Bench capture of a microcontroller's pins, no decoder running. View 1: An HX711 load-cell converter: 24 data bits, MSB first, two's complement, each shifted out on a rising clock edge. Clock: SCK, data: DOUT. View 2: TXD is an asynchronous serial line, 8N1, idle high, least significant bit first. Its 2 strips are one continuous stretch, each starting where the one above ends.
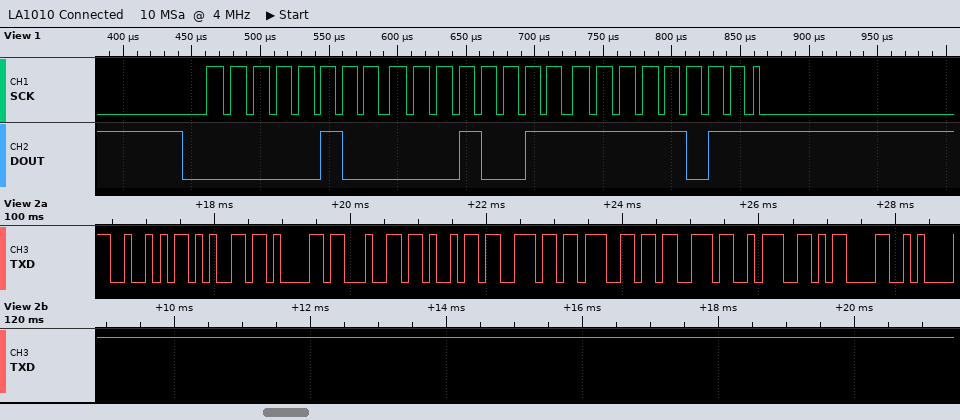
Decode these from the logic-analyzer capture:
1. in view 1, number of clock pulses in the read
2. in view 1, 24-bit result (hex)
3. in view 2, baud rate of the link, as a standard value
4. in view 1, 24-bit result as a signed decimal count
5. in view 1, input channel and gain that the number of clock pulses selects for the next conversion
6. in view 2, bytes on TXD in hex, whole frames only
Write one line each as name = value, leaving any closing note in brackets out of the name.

in view 1, number of clock pulses in the read = 25
in view 1, 24-bit result = 0x0413FB
in view 2, baud rate of the link, as a standard value = 9600 baud
in view 1, 24-bit result as a signed decimal count = 267259
in view 1, input channel and gain that the number of clock pulses selects for the next conversion = channel A, gain 128
in view 2, bytes on TXD in hex, whole frames only = 52 65 61 64 69 6E 67 73 3A 0D 0A
